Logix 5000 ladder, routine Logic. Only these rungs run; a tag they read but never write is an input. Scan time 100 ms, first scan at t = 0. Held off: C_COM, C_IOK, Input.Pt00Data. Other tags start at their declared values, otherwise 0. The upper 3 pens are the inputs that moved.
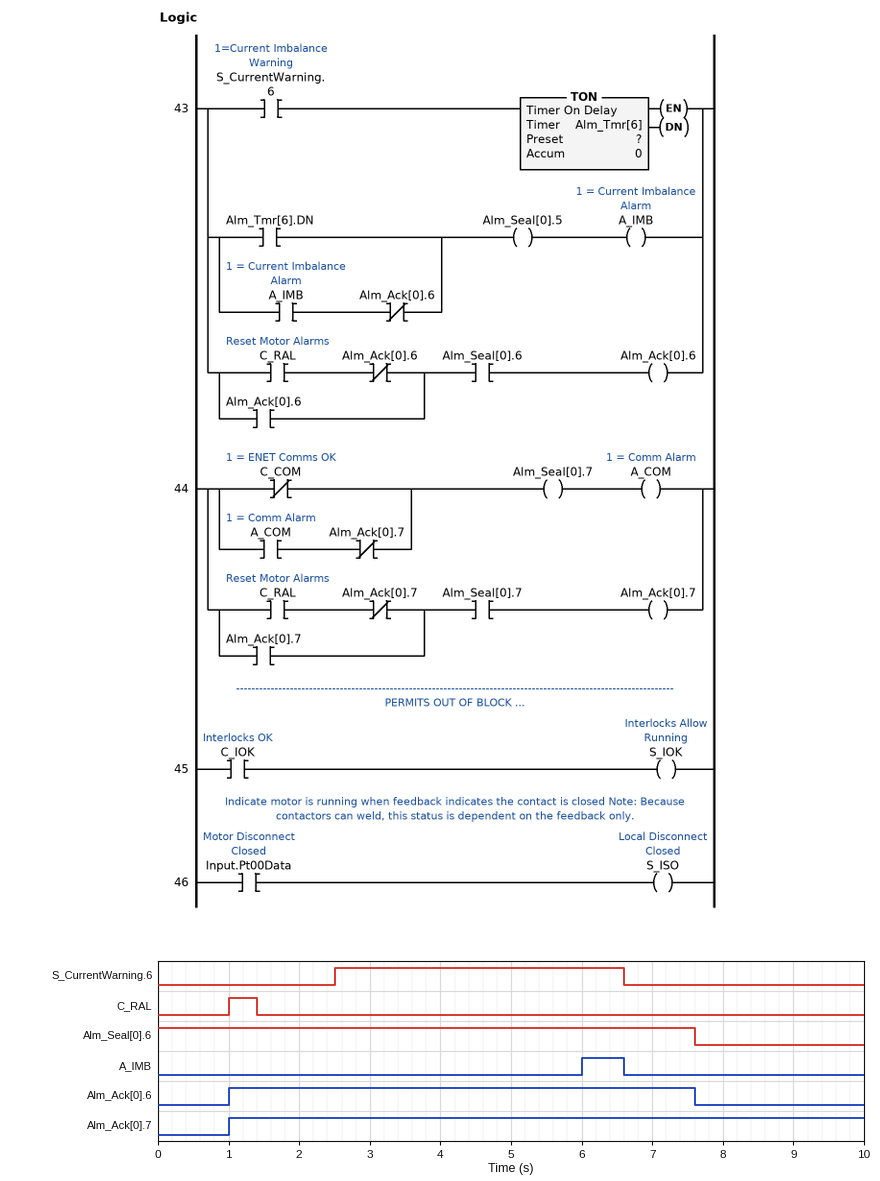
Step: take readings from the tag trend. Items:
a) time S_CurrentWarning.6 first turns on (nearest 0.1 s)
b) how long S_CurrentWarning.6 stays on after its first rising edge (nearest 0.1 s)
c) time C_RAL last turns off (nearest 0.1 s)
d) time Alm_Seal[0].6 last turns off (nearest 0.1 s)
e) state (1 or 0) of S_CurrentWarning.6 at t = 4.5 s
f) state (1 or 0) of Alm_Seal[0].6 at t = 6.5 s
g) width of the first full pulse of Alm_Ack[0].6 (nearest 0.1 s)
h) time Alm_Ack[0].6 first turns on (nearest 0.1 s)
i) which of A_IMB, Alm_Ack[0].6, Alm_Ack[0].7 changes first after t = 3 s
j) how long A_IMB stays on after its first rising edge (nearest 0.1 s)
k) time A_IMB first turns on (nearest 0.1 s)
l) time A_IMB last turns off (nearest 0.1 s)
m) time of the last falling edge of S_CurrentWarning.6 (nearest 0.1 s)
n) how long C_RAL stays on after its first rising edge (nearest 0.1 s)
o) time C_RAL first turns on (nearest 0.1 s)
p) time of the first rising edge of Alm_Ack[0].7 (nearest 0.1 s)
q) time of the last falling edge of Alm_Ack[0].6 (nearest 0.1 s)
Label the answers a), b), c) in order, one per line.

a) 2.5 s
b) 4.1 s
c) 1.4 s
d) 7.6 s
e) 1
f) 1
g) 6.6 s
h) 1.0 s
i) A_IMB
j) 0.6 s
k) 6.0 s
l) 6.6 s
m) 6.6 s
n) 0.4 s
o) 1.0 s
p) 1.0 s
q) 7.6 s
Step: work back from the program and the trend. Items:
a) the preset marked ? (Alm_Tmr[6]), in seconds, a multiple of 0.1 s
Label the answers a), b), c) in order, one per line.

a) 3.5 s
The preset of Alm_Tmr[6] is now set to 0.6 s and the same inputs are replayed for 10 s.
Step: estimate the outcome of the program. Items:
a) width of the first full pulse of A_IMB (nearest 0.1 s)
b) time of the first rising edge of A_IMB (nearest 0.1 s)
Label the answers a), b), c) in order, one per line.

a) 3.5 s
b) 3.1 s
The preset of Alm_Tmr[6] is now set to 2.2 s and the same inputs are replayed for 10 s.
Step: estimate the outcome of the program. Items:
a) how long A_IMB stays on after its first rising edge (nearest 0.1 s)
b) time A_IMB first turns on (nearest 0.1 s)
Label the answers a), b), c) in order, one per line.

a) 1.9 s
b) 4.7 s
